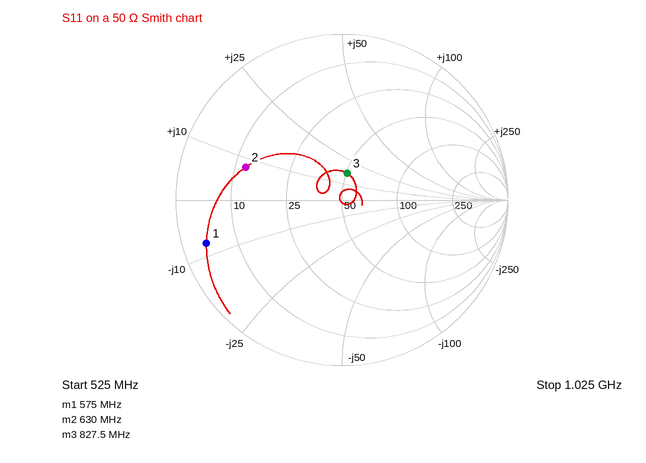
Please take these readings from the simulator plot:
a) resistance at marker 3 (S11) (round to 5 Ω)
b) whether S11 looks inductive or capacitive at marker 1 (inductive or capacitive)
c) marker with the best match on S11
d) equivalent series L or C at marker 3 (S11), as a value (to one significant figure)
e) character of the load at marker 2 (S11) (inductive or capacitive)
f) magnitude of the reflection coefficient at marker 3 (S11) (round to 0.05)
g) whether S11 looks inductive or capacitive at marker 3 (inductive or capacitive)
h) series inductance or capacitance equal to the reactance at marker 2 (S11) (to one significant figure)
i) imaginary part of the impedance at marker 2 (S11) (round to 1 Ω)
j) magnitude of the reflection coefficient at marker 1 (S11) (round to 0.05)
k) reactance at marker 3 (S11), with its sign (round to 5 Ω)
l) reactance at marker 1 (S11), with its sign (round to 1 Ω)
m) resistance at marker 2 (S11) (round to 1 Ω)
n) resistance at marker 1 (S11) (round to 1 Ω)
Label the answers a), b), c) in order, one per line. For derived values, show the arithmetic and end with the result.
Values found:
a) 50 Ω
b) capacitive
c) marker 3
d) L = 15 Ω/(2π × 827.5 MHz) ≈ 3 nH
e) inductive
f) 0.15
g) inductive
h) L = 8 Ω/(2π × 630 MHz) ≈ 2 nH
i) +8 Ω
j) 0.85
k) +15 Ω
l) -8 Ω
m) 12 Ω
n) 4 Ω
